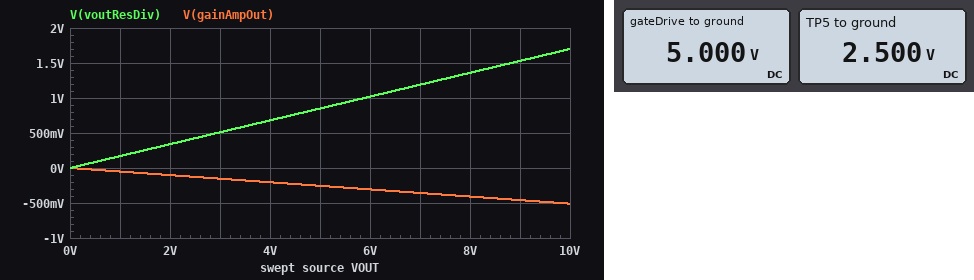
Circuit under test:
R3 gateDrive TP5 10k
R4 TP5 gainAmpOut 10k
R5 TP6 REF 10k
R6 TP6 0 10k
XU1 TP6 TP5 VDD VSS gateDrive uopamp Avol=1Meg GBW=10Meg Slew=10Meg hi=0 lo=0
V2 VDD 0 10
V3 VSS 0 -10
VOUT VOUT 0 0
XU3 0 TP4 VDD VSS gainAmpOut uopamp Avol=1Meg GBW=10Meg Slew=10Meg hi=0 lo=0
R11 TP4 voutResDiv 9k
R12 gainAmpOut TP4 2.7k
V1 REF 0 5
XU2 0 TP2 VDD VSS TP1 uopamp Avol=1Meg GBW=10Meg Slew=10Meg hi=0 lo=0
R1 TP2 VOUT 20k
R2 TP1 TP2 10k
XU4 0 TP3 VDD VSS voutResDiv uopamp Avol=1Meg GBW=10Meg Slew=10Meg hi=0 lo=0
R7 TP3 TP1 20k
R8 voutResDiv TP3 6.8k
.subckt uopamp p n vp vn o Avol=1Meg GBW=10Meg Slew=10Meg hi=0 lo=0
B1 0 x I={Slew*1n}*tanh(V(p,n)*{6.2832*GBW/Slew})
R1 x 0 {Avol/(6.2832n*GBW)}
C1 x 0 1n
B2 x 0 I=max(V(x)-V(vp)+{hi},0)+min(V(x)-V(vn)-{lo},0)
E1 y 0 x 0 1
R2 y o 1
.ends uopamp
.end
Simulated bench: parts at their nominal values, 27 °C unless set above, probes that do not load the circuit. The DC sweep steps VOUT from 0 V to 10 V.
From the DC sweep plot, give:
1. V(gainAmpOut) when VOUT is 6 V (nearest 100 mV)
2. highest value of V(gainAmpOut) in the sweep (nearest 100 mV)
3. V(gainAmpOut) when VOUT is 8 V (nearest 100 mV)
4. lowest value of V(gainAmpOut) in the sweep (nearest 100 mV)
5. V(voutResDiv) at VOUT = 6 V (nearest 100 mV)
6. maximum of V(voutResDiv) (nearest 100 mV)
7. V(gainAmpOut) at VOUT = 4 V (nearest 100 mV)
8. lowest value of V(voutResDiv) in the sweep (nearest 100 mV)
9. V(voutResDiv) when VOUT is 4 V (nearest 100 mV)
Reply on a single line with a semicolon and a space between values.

-300 mV; 0 V; -400 mV; -500 mV; 1.0 V; 1.7 V; -200 mV; 0 V; 700 mV
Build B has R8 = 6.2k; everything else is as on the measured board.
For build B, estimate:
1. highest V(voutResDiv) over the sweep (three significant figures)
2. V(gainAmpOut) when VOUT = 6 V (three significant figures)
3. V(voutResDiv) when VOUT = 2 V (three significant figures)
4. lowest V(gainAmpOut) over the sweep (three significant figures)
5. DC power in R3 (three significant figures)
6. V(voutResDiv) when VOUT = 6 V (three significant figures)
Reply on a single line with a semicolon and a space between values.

1.55 V; -279 mV; 310 mV; -465 mV; 625 µW; 930 mV
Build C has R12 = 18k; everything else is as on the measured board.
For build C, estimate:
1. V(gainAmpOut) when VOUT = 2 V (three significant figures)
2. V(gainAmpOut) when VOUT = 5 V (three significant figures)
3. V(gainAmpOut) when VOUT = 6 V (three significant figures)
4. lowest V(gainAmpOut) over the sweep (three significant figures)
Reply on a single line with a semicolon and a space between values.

-680 mV; -1.70 V; -2.04 V; -3.40 V
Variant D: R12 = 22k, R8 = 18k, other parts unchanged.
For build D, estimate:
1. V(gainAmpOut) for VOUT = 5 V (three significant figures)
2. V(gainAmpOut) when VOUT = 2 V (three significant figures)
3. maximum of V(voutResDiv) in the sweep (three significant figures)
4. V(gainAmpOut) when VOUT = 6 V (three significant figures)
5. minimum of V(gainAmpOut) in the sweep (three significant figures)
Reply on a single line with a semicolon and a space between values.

-5.50 V; -2.20 V; 4.50 V; -6.60 V; -10.0 V
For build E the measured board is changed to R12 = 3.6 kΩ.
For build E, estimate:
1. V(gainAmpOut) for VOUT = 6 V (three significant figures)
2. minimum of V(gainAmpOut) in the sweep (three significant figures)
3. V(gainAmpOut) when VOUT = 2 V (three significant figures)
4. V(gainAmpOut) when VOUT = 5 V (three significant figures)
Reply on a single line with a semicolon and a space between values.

-408 mV; -680 mV; -136 mV; -340 mV
